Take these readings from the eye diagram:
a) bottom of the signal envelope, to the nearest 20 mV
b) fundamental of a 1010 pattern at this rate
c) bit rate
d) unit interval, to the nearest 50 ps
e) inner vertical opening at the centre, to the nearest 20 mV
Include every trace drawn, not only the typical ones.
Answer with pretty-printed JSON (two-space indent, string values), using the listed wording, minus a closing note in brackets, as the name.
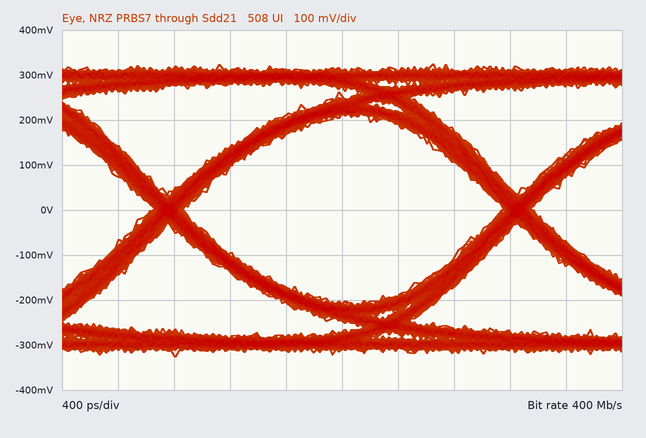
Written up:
{
  "bottom of the signal envelope, to the nearest 20 mV": "-320 mV",
  "fundamental of a 1010 pattern at this rate": "200 MHz",
  "bit rate": "400 Mb/s",
  "unit interval, to the nearest 50 ps": "2.50 ns",
  "inner vertical opening at the centre, to the nearest 20 mV": "420 mV"
}
